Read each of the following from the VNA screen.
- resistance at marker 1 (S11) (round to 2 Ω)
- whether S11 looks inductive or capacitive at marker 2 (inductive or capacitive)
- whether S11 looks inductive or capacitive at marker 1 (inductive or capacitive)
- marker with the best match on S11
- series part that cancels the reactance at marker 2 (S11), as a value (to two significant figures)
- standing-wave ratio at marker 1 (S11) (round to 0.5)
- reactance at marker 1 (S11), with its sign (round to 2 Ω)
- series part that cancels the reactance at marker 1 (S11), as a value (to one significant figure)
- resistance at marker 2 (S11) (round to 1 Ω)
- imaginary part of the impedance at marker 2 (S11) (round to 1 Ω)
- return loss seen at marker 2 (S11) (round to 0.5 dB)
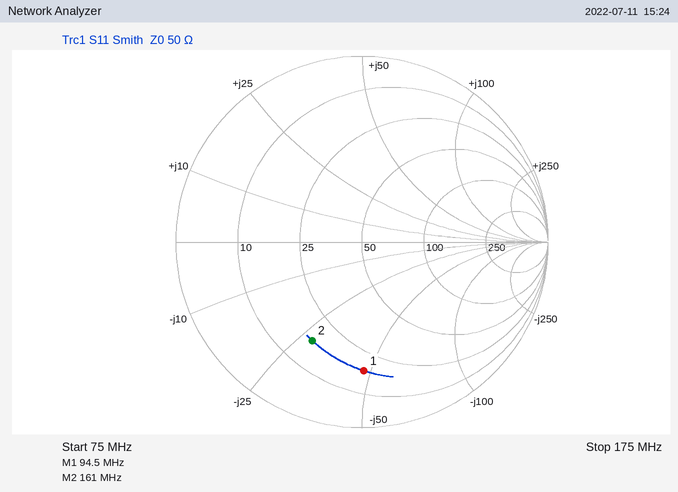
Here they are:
18 Ω
capacitive
capacitive
marker 2
28 nH
5.5
-48 Ω
80 nH
17 Ω
-28 Ω
4.5 dB
